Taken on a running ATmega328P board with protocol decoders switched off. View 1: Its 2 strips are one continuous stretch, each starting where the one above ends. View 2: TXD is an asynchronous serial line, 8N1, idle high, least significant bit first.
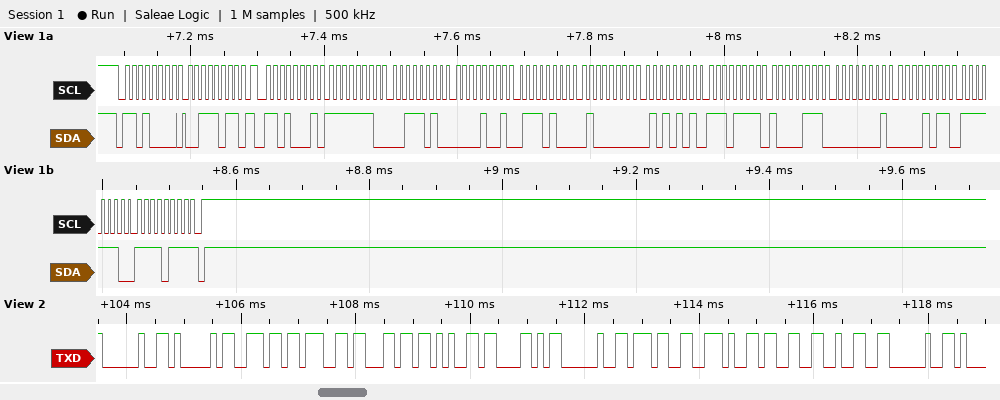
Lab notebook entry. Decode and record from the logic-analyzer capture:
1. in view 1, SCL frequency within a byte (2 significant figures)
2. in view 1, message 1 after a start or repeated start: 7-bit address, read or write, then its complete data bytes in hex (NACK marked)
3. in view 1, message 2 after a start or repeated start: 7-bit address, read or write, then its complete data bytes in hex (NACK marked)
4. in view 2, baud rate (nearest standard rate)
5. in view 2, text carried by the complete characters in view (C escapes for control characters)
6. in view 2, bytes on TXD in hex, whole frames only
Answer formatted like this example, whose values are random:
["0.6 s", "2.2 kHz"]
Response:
["100 kHz", "0x68 write: 3B", "0x68 read: FE 3A 09 74 40 55 EF 87 01 0B FE F7 NACK", "9600 baud", "\" AngleX 7.32 \"", "20 41 6E 67 6C 65 58 20 37 2E 33 32 20"]
